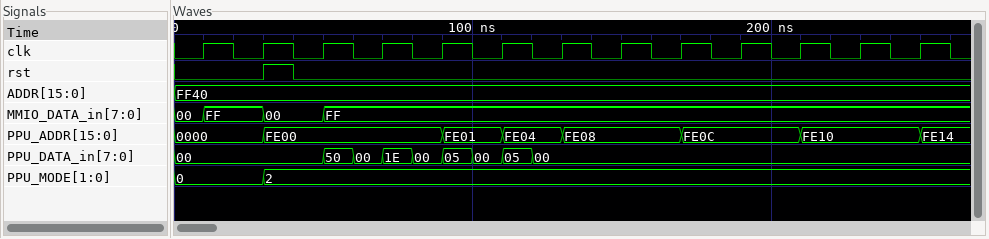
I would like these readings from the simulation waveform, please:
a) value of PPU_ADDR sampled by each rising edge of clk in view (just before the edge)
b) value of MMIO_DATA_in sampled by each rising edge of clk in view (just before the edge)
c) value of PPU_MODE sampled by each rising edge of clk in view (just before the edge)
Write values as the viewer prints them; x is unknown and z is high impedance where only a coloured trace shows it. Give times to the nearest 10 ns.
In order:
0000, 0000, FE00, FE00, FE00, FE01, FE04, FE08, FE08, FE0C, FE0C, FE10, FE10
00, FF, 00, FF, FF, FF, FF, FF, FF, FF, FF, FF, FF
0, 0, 2, 2, 2, 2, 2, 2, 2, 2, 2, 2, 2
